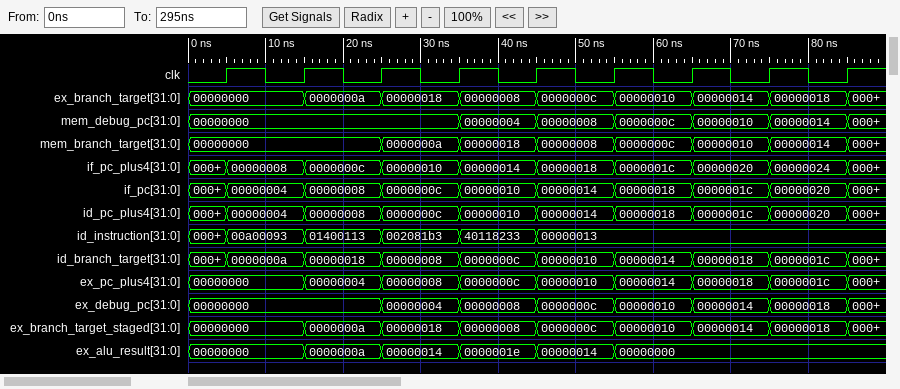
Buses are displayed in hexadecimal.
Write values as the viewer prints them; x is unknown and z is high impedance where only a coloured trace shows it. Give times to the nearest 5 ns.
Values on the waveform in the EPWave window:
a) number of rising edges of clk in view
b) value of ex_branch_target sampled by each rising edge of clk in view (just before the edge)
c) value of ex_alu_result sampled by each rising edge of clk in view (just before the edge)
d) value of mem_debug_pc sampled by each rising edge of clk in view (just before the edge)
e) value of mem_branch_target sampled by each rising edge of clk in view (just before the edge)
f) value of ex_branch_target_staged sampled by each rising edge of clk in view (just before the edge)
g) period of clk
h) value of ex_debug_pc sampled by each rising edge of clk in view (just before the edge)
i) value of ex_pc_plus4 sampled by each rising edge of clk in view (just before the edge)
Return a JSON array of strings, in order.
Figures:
["9", "00000000, 00000000, 0000000a, 00000018, 00000008, 0000000c, 00000010, 00000014, 00000018", "00000000, 00000000, 0000000a, 00000014, 0000001e, 00000014, 00000000, 00000000, 00000000", "00000000, 00000000, 00000000, 00000000, 00000004, 00000008, 0000000c, 00000010, 00000014", "00000000, 00000000, 00000000, 0000000a, 00000018, 00000008, 0000000c, 00000010, 00000014", "00000000, 00000000, 0000000a, 00000018, 00000008, 0000000c, 00000010, 00000014, 00000018", "10 ns", "00000000, 00000000, 00000000, 00000004, 00000008, 0000000c, 00000010, 00000014, 00000018", "00000000, 00000000, 00000004, 00000008, 0000000c, 00000010, 00000014, 00000018, 0000001c"]
